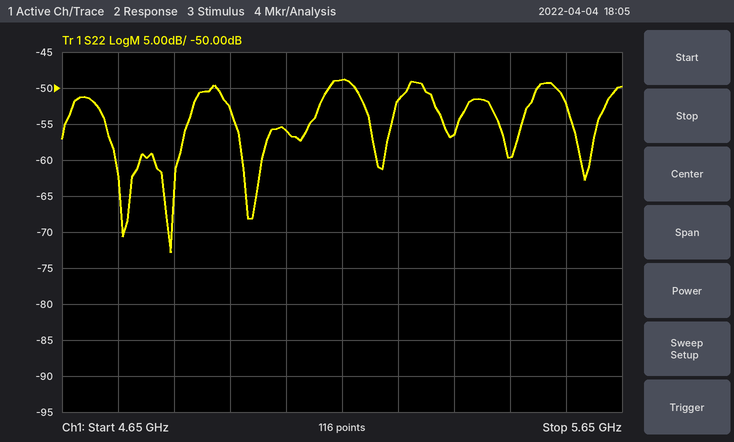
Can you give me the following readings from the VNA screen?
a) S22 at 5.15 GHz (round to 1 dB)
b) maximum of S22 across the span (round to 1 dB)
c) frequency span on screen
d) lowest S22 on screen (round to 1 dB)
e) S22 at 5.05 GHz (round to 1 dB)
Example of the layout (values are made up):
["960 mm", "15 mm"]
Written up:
["-49 dB", "-49 dB", "1 GHz", "-73 dB", "-56 dB"]
